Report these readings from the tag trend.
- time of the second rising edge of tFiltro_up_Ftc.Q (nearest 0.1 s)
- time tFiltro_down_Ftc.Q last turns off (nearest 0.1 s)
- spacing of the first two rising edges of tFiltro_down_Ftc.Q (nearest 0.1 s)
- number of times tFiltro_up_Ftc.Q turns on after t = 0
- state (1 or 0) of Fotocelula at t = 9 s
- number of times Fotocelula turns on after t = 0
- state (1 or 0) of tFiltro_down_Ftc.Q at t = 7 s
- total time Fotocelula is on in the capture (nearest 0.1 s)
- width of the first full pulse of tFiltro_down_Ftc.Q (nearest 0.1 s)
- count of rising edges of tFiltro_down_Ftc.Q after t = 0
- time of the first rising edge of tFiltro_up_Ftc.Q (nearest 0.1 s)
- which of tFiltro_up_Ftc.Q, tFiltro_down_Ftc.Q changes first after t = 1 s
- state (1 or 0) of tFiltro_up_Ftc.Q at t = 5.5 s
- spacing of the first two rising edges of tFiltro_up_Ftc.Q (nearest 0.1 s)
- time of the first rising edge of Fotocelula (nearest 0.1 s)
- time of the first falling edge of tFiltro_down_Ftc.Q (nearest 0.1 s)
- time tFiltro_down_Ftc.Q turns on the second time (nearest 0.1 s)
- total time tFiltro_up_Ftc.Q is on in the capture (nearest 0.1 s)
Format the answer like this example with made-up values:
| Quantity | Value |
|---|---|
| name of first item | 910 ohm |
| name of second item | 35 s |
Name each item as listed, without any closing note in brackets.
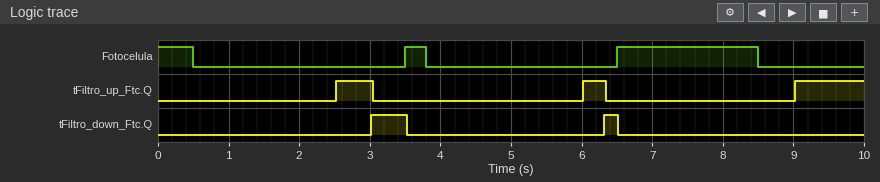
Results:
| Quantity | Value |
|---|---|
| time of the second rising edge of tFiltro_up_Ftc.Q | 6.0 s |
| time tFiltro_down_Ftc.Q last turns off | 6.5 s |
| spacing of the first two rising edges of tFiltro_down_Ftc.Q | 3.3 s |
| number of times tFiltro_up_Ftc.Q turns on after t = 0 | 3 |
| state (1 or 0) of Fotocelula at t = 9 s | 0 |
| number of times Fotocelula turns on after t = 0 | 2 |
| state (1 or 0) of tFiltro_down_Ftc.Q at t = 7 s | 0 |
| total time Fotocelula is on in the capture | 2.8 s |
| width of the first full pulse of tFiltro_down_Ftc.Q | 0.5 s |
| count of rising edges of tFiltro_down_Ftc.Q after t = 0 | 2 |
| time of the first rising edge of tFiltro_up_Ftc.Q | 2.5 s |
| which of tFiltro_up_Ftc.Q, tFiltro_down_Ftc.Q changes first after t = 1 s | tFiltro_up_Ftc.Q |
| state (1 or 0) of tFiltro_up_Ftc.Q at t = 5.5 s | 0 |
| spacing of the first two rising edges of tFiltro_up_Ftc.Q | 3.5 s |
| time of the first rising edge of Fotocelula | 3.5 s |
| time of the first falling edge of tFiltro_down_Ftc.Q | 3.5 s |
| time tFiltro_down_Ftc.Q turns on the second time | 6.3 s |
| total time tFiltro_up_Ftc.Q is on in the capture | 1.8 s |
